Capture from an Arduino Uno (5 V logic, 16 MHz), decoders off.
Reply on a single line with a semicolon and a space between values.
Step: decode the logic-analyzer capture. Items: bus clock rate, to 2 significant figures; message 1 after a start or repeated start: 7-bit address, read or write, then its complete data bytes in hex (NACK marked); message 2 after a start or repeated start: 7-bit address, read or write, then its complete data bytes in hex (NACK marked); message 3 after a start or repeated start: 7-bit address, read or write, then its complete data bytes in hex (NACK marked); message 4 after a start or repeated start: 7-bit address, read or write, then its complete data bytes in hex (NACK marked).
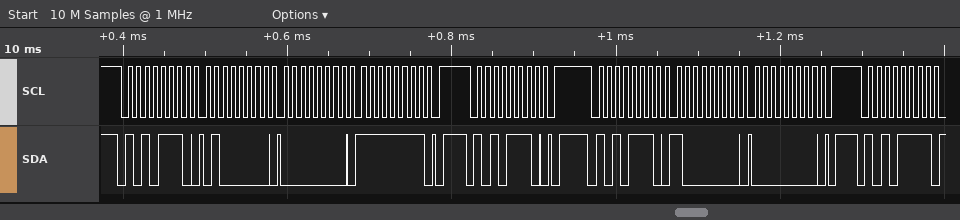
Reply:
100 kHz; 0x57 write: 40 00 FF; 0x57 write; 0x57 write: 80 00; 0x57 read
